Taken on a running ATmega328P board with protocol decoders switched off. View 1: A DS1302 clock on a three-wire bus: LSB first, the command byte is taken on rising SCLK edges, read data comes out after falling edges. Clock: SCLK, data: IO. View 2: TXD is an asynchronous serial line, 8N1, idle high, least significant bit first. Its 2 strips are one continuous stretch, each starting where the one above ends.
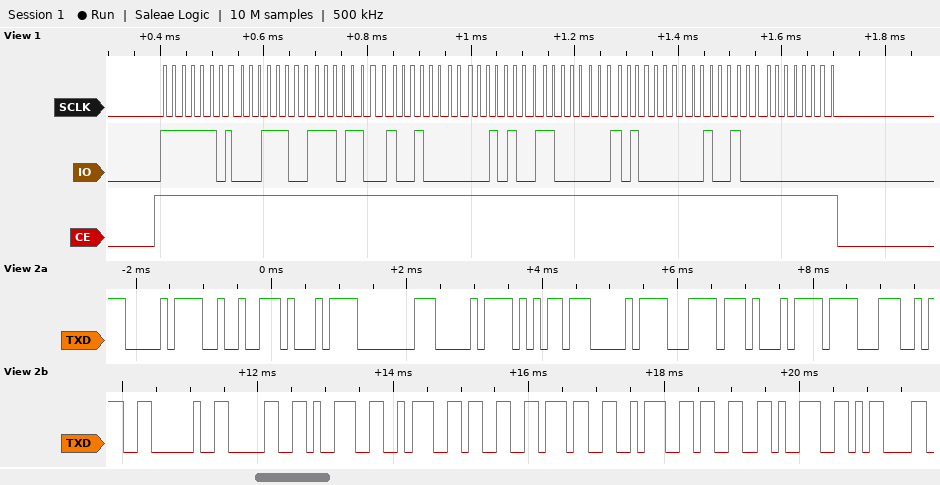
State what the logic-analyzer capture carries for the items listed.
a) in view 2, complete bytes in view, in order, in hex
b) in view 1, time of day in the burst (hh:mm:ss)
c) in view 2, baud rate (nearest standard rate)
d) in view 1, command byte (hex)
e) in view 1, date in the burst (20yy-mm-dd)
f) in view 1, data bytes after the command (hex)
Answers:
D0 92 D1 80 D0 B5 D0 BC D1 8F 3A 20 30 39 3A 33 37 3A 33 39 0D
09:37:38
9600 baud
0xBF
2024-03-28
38 37 09 28 03 05 24 00
